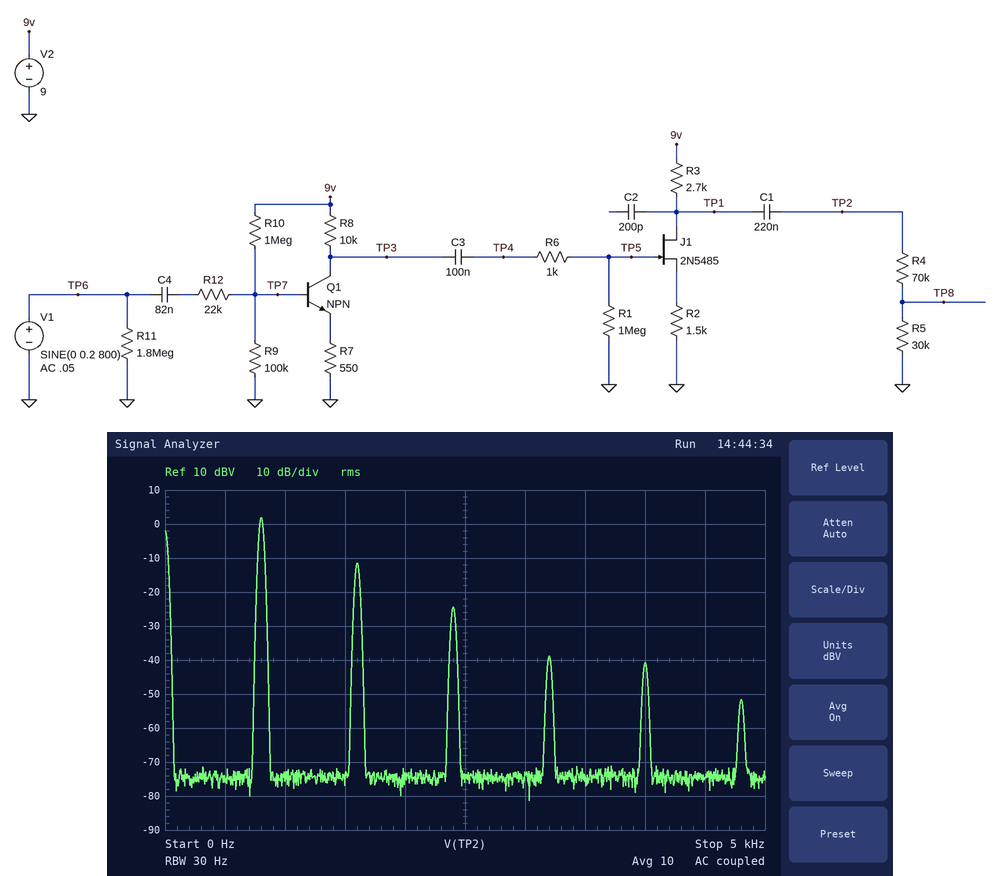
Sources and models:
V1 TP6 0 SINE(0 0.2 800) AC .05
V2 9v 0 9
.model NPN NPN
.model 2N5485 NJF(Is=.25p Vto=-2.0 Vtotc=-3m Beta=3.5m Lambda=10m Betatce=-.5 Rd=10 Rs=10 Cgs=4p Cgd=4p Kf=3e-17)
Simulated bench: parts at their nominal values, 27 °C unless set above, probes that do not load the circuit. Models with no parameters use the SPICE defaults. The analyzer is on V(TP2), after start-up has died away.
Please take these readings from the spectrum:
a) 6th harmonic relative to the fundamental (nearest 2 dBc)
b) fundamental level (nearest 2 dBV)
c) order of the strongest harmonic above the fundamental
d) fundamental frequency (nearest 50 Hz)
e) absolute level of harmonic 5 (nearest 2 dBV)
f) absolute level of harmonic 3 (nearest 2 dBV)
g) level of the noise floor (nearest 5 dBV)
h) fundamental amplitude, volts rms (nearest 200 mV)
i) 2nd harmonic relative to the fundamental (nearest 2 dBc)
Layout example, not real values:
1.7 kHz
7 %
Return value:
-54 dBc
2 dBV
2
800 Hz
-40 dBV
-24 dBV
-75 dBV
1.2 V
-14 dBc
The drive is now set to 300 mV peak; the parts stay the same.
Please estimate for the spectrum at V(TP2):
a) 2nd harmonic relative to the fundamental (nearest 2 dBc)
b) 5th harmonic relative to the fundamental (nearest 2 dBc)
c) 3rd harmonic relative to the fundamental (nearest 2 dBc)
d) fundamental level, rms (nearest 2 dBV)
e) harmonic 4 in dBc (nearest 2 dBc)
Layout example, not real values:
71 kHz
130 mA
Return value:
-10 dBc
-44 dBc
-24 dBc
4 dBV
-26 dBc
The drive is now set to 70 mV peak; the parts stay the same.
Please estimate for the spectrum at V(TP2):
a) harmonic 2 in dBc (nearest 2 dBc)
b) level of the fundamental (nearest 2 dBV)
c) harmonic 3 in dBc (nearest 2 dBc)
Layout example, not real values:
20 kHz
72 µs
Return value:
-26 dBc
-6 dBV
-42 dBc
